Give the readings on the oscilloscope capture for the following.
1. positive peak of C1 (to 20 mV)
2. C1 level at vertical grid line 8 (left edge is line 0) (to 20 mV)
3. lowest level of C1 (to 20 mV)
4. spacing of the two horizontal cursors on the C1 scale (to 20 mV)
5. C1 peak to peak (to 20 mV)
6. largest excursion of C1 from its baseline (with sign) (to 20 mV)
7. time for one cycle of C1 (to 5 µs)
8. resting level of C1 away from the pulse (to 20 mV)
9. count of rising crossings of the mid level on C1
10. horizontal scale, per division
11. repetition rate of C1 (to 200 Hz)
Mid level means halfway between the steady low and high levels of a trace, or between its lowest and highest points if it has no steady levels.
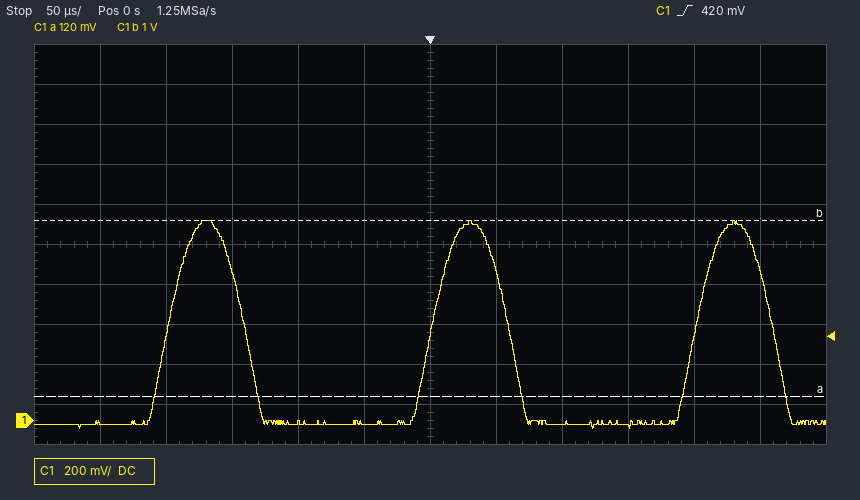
1.00 V
-20 mV
-40 mV
880 mV
1.04 V
+1.02 V
200 µs
-20 mV
3
50 µs
5.0 kHz
